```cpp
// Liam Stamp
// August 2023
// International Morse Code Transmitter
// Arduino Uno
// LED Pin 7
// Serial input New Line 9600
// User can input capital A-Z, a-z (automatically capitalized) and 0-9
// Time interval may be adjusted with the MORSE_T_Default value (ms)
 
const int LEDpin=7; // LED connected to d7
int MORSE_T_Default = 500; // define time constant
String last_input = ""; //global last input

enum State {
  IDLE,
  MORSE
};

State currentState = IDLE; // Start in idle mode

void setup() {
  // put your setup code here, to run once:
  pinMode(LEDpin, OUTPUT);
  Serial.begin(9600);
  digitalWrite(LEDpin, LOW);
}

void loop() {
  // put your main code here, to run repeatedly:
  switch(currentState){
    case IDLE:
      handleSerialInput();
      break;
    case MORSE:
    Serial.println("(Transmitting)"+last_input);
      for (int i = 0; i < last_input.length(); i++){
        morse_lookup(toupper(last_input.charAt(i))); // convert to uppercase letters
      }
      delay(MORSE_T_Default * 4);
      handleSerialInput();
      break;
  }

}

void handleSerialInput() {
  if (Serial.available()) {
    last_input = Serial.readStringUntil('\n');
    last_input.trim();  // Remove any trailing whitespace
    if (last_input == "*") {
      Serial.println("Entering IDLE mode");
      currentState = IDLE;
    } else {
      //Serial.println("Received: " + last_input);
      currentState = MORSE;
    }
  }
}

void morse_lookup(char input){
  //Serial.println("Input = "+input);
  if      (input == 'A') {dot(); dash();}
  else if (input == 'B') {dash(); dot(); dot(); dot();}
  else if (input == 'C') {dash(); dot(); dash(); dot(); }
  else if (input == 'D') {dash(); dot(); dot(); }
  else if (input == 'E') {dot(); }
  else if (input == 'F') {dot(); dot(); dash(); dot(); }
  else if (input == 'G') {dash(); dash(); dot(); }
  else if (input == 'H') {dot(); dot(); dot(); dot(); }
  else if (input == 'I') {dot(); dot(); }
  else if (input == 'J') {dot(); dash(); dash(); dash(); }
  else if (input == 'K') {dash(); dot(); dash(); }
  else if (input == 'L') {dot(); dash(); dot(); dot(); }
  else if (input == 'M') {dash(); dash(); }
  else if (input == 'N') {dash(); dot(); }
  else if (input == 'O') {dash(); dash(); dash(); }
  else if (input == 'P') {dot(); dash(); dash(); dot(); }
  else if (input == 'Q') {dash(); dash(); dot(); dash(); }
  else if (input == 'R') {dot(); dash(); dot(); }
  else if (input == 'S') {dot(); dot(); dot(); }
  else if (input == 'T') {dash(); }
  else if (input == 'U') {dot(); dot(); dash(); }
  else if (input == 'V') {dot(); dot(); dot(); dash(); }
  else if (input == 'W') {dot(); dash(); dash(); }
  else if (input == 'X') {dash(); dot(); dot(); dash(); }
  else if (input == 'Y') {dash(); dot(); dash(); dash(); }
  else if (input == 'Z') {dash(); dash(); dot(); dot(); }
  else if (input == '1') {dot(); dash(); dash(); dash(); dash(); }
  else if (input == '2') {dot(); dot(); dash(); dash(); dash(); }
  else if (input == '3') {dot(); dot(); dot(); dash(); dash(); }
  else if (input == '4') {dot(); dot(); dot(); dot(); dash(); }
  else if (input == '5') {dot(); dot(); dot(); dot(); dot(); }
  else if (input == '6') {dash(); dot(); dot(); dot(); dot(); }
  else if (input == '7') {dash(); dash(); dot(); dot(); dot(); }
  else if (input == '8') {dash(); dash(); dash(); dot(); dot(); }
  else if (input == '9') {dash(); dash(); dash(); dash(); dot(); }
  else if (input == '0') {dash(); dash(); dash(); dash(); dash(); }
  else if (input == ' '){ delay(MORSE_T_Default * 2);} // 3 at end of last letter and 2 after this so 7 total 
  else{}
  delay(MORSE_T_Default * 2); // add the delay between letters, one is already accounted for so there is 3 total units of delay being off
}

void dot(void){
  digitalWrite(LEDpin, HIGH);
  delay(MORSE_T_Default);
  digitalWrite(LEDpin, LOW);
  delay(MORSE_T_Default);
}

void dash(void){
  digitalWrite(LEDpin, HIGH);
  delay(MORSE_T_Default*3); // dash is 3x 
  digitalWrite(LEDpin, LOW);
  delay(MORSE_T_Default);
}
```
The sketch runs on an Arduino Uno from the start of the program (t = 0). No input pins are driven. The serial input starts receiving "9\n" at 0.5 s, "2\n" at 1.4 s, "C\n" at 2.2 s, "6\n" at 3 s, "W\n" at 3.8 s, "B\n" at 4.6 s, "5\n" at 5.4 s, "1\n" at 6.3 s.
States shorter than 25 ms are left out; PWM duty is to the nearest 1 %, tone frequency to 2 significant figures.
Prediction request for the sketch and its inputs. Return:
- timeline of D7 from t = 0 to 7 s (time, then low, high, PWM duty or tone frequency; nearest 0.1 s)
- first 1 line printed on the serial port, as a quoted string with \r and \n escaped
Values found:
0 s low; 0.5 s high; 2 s low; 2.5 s high; 4 s low; 4.5 s high; 6 s low; 6.5 s high
"(Transmitting)9\r\n"
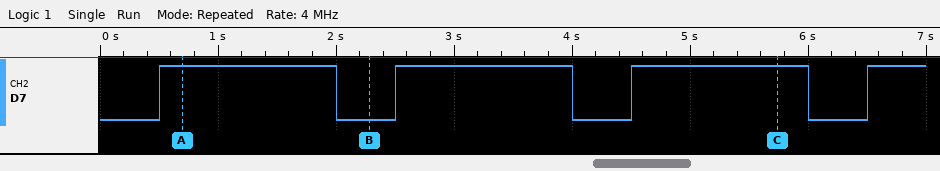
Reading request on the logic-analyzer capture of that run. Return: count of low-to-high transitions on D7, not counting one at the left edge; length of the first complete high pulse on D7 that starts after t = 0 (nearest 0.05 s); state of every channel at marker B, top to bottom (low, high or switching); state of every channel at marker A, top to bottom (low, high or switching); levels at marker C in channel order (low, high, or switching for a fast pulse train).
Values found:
4
1.50 s
D7 low
D7 high
D7 high
